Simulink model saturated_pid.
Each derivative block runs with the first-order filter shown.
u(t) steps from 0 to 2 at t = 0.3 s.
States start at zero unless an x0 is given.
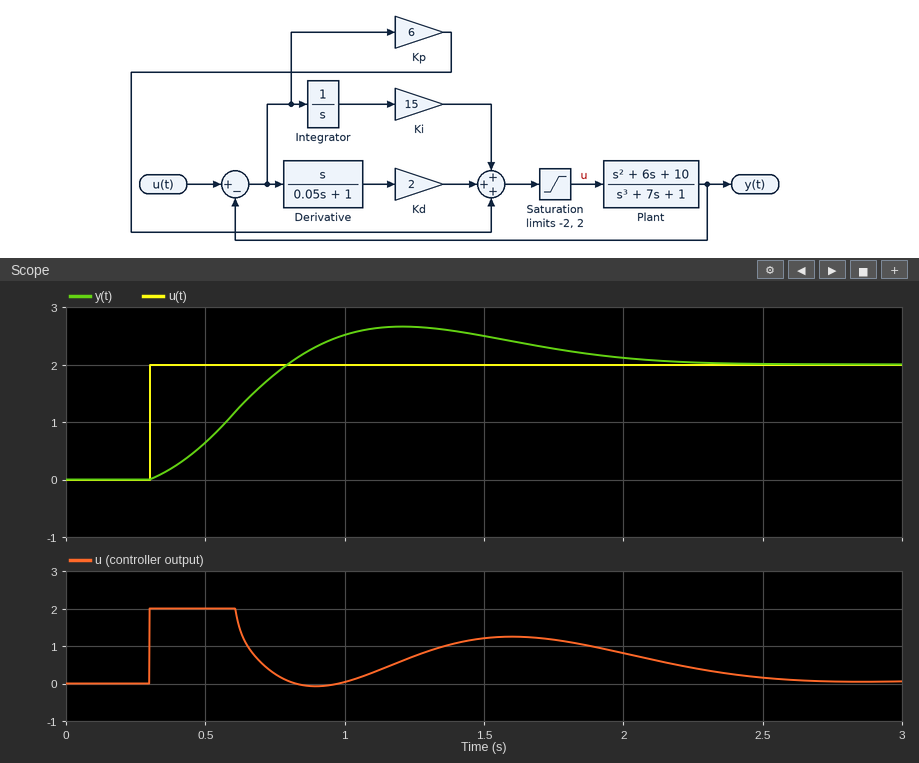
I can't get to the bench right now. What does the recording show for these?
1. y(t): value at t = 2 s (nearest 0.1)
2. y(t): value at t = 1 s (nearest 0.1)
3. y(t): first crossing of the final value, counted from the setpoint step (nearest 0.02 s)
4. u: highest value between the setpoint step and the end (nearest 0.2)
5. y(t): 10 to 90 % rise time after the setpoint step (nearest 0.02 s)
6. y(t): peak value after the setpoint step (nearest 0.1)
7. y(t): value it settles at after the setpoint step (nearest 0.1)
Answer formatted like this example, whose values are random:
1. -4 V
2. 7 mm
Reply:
1. 2.1
2. 2.5
3. 0.50 s
4. 2.0
5. 0.36 s
6. 2.7
7. 2.0
